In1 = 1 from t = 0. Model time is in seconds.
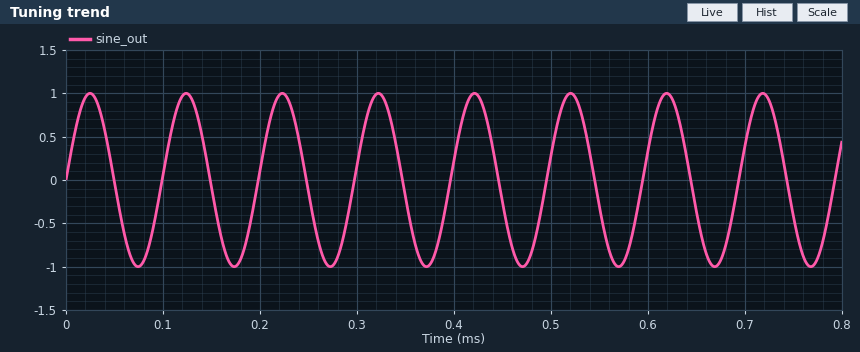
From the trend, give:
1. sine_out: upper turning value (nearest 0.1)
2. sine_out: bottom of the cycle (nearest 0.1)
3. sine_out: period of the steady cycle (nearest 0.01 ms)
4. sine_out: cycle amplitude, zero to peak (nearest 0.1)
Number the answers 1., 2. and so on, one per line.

1. 1.0
2. -1.0
3. 0.10 ms
4. 1.0
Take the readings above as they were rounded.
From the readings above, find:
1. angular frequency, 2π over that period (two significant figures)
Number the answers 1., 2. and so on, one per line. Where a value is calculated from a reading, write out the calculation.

1. 2π / 0.1 = 63 rad/ms
